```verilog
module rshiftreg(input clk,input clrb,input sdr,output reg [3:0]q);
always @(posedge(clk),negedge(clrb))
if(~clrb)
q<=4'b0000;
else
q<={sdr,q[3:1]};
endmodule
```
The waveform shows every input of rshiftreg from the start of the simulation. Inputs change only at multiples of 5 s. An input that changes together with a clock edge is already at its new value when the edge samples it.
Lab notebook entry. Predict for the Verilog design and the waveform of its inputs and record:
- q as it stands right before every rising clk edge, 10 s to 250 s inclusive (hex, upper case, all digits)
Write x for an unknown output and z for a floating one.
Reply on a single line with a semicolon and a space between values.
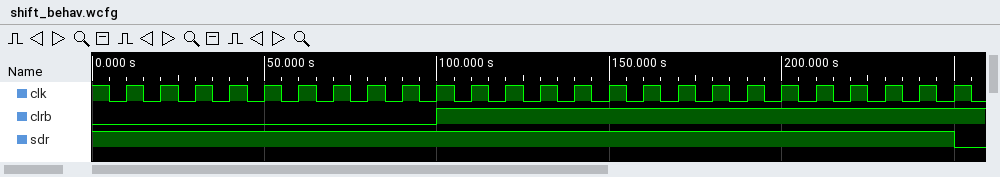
0, 0, 0, 0, 0, 0, 0, 0, 0, 0, 8, C, E, F, F, F, F, F, F, F, F, F, F, F, F
